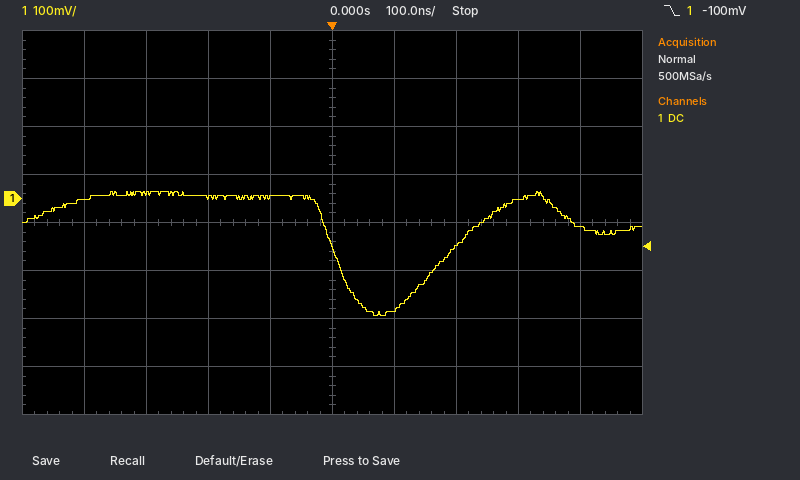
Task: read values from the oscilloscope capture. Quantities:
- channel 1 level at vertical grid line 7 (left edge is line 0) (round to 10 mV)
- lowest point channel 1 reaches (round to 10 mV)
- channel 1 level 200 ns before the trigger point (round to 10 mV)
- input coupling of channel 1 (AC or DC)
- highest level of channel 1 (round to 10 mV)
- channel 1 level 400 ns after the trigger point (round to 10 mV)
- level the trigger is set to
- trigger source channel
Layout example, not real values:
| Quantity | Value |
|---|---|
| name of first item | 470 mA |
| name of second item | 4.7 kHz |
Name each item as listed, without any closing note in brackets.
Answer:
| Quantity | Value |
|---|---|
| channel 1 level at vertical grid line 7 (left edge is line 0) | -100 mV |
| lowest point channel 1 reaches | -240 mV |
| channel 1 level 200 ns before the trigger point | 0 mV |
| input coupling of channel 1 | DC |
| highest level of channel 1 | 10 mV |
| channel 1 level 400 ns after the trigger point | -60 mV |
| level the trigger is set to | -100 mV |
| trigger source channel | channel 1 |
